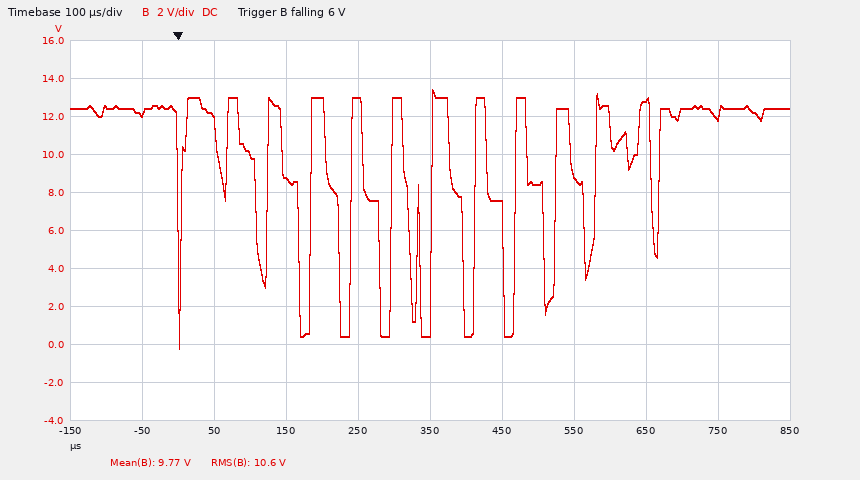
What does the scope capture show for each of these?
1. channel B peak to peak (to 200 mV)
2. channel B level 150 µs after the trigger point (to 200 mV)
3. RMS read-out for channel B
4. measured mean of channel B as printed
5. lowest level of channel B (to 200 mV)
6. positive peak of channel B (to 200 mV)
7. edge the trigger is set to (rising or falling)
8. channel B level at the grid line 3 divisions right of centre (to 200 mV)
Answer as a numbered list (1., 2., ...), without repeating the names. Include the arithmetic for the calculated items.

1. 13.4 V − (-200 mV) = 13.6 V
2. 8.8 V
3. 10.6 V
4. 9.77 V
5. -200 mV
6. 13.4 V
7. falling
8. 12.8 V
